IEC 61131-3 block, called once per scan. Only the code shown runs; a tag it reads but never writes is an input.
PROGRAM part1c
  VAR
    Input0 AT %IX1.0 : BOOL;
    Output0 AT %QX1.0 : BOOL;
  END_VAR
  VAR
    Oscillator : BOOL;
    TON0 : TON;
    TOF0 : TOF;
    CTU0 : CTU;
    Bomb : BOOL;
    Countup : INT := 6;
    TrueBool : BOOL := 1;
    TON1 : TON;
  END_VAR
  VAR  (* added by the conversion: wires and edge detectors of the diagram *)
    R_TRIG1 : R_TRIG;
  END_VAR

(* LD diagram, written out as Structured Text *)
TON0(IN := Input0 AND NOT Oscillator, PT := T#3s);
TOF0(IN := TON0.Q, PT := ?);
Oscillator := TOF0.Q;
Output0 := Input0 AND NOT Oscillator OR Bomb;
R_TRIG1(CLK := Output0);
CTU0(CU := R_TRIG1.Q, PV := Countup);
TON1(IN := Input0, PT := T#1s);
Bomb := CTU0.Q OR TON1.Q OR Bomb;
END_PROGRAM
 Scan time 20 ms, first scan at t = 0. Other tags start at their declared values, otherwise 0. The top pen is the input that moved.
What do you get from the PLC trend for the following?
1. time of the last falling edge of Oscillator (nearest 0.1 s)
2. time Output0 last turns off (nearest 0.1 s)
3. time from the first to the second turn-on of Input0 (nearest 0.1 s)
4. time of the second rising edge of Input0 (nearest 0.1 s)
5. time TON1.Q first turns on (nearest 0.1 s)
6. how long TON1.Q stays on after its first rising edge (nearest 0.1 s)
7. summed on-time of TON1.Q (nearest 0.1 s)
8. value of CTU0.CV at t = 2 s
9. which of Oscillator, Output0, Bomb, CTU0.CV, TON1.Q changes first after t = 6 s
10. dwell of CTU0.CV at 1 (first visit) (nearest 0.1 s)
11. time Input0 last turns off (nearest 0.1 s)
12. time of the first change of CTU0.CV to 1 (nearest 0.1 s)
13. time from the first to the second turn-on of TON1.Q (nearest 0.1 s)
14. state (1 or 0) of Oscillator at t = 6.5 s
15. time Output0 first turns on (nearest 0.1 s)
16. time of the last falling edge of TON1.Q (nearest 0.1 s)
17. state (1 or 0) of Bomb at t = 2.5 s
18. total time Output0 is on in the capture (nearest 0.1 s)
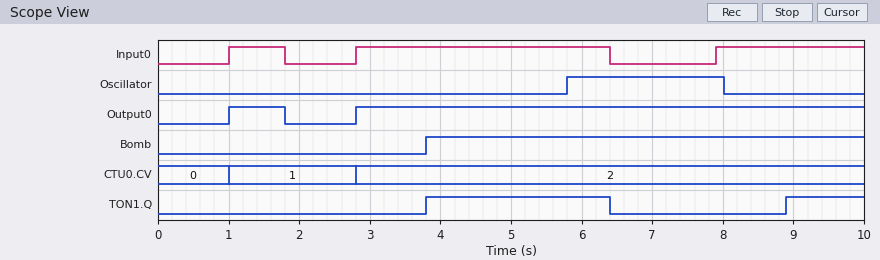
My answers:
8.0 s
1.8 s
1.8 s
2.8 s
3.8 s
2.6 s
3.7 s
1
TON1.Q
1.8 s
6.4 s
1.0 s
5.1 s
1
1.0 s
6.4 s
0
8.0 s
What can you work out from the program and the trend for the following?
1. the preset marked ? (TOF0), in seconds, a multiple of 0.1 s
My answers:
2.2 s
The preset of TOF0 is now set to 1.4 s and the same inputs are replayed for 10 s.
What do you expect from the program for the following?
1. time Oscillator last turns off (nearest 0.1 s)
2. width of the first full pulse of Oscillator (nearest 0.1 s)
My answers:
7.2 s
1.4 s
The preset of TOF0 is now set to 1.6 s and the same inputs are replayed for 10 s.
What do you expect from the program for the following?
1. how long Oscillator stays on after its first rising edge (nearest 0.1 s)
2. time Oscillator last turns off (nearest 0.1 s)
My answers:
1.6 s
7.4 s
